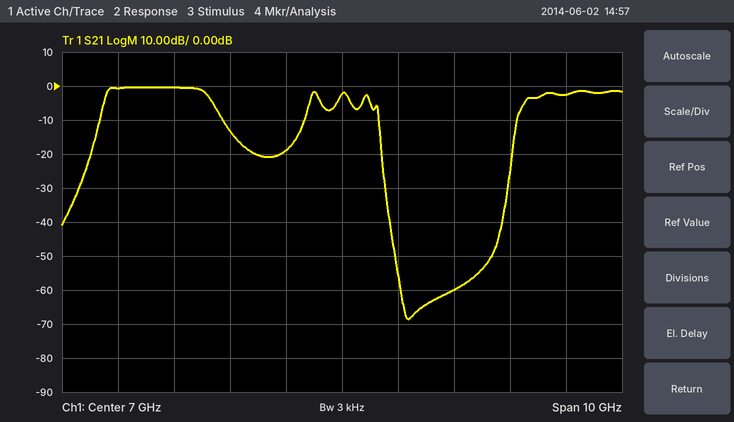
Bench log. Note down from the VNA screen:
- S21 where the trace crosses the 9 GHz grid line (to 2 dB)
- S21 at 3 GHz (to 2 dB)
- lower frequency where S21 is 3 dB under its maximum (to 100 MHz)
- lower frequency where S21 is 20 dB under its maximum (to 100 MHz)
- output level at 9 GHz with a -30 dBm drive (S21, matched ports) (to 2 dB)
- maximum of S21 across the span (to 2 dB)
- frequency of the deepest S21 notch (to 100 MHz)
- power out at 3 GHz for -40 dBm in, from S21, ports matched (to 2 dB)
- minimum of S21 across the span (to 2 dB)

-60 dB
0 dB
2.8 GHz
2.5 GHz
-90 dBm
0 dB
8.2 GHz
-40 dBm
-68 dB
